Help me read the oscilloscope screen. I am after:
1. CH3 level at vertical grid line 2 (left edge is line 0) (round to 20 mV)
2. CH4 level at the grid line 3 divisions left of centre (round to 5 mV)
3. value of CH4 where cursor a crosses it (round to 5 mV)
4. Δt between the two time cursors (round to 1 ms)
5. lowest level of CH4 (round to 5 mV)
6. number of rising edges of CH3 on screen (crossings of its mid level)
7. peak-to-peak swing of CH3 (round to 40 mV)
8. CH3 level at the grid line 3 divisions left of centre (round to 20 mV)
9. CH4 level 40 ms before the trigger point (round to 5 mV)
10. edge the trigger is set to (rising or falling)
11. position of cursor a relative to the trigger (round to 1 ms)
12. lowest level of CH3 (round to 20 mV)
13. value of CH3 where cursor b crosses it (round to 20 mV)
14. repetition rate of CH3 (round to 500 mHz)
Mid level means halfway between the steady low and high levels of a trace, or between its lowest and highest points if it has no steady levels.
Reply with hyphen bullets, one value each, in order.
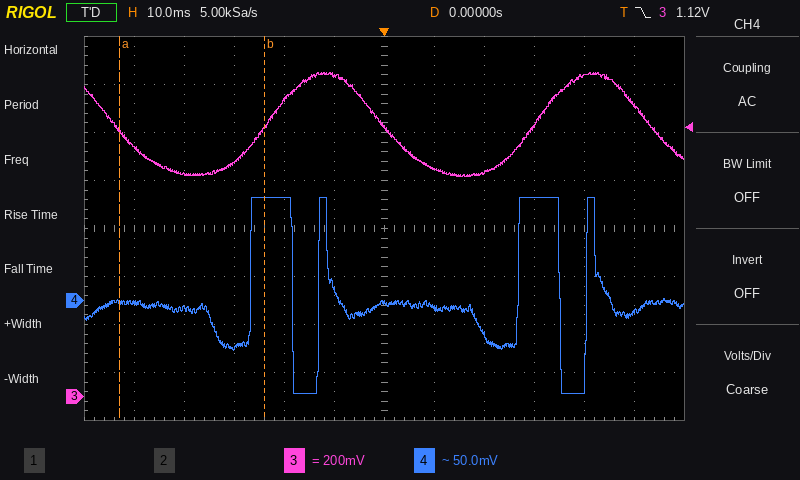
- 920 mV
- -50 mV
- 0 mV
- 29 ms
- -95 mV
- 2
- 440 mV
- 980 mV
- -10 mV
- falling
- -53 ms
- 920 mV
- 1.12 V
- 18.5 Hz
